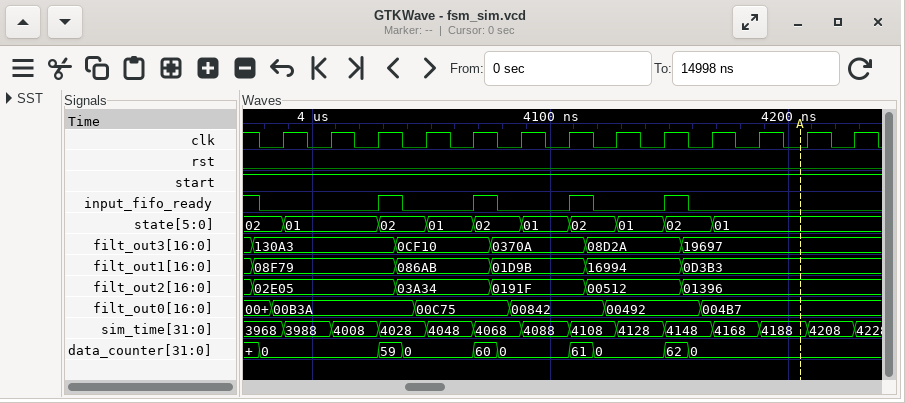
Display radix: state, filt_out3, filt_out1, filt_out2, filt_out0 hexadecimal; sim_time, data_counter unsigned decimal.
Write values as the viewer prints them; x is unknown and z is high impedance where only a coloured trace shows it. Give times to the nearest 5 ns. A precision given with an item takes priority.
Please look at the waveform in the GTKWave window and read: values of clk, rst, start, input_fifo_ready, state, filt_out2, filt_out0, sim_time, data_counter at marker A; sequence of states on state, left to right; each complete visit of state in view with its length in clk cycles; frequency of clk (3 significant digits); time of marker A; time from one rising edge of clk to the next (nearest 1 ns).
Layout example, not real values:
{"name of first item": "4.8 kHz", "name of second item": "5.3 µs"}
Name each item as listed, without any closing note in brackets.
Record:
{"values of clk, rst, start, input_fifo_ready, state, filt_out2, filt_out0, sim_time, data_counter at marker A": "clk=0, rst=0, start=1, input_fifo_ready=0, state=01, filt_out2=01396, filt_out0=004B7, sim_time=4188, data_counter=0", "sequence of states on state, left to right": "02, 01, 02, 01, 02, 01, 02, 01, 02, 01", "each complete visit of state in view with its length in clk cycles": "01: 2, 02: 1, 01: 1, 02: 1, 01: 1, 02: 1, 01: 1, 02: 1", "frequency of clk": "50.0 MHz", "time of marker A": "4205 ns", "time from one rising edge of clk to the next": "20 ns"}
